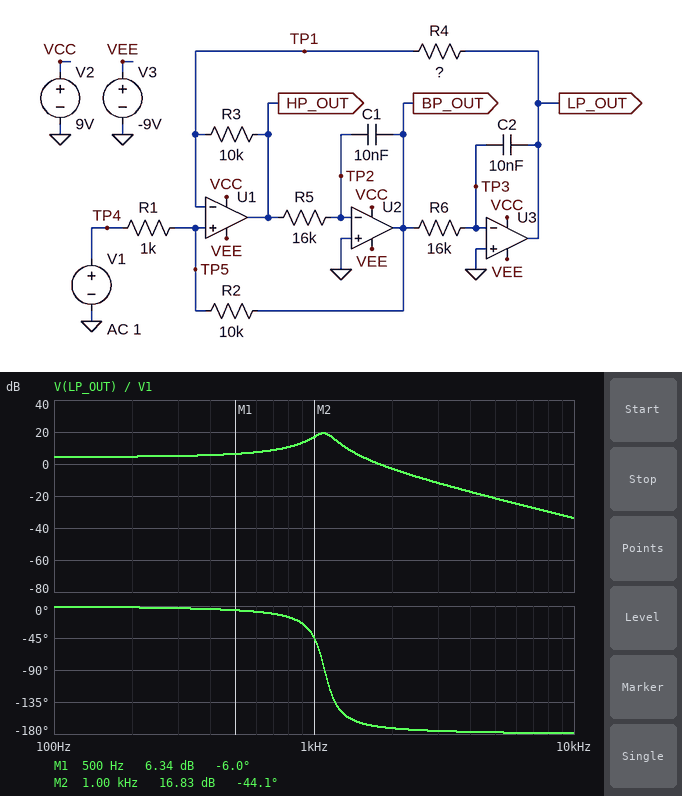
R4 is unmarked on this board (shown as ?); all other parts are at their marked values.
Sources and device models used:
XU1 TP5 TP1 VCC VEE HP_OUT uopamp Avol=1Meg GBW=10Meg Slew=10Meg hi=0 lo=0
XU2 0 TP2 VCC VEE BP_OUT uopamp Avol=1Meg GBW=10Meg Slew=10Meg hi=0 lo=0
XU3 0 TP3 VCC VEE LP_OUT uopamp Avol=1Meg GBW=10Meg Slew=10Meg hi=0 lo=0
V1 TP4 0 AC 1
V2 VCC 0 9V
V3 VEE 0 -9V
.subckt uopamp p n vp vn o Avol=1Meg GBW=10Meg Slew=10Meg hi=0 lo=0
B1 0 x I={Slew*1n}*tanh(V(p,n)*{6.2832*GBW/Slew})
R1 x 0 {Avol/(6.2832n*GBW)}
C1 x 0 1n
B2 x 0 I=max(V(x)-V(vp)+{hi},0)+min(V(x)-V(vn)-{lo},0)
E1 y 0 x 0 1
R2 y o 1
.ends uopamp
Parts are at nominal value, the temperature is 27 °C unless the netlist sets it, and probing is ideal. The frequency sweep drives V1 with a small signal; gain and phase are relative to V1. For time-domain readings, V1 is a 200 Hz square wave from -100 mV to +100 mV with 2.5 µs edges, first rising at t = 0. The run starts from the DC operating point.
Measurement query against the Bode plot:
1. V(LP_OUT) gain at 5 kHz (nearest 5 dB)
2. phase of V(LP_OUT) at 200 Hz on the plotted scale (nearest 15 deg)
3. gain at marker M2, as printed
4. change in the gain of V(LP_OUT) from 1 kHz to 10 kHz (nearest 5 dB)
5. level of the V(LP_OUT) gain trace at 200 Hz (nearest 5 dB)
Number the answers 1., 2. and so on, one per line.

1. -20 dB
2. 0 deg
3. 16.83 dB
4. -50 dB
5. 5 dB
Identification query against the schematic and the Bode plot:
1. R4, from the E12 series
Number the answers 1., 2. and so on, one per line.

1. 8.2 kΩ
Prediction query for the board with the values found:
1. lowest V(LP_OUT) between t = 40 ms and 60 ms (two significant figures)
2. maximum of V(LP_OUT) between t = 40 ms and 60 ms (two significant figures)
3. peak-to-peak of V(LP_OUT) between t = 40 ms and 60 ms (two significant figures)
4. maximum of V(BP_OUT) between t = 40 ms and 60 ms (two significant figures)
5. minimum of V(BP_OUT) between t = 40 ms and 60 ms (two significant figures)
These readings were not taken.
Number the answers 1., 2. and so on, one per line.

1. -420 mV
2. 420 mV
3. 840 mV
4. 330 mV
5. -330 mV
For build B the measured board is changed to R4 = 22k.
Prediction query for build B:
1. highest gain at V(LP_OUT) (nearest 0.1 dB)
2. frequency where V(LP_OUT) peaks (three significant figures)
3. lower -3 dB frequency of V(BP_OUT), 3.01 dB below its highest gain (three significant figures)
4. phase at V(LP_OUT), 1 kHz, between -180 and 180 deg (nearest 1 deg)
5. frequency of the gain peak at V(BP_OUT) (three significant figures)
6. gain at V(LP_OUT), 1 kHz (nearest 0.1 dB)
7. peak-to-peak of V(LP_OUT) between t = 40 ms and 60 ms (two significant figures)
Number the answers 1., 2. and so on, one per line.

1. 23.5 dB
2. 664 Hz
3. 608 Hz
4. -167 deg
5. 671 Hz
6. 7.3 dB
7. 1.6 V
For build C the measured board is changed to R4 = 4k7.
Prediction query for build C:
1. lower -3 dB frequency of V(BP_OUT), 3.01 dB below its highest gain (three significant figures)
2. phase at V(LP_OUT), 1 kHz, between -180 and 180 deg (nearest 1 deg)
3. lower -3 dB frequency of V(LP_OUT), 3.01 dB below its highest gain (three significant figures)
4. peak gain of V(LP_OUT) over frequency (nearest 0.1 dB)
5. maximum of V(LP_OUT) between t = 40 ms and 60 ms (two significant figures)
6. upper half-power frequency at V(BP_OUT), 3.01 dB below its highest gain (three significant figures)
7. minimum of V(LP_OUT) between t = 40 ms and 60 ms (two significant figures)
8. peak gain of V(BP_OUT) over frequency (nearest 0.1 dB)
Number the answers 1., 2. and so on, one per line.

1. 1.32 kHz
2. -14 deg
3. 1.29 kHz
4. 16.8 dB
5. 350 mV
6. 1.60 kHz
7. -350 mV
8. 20.0 dB
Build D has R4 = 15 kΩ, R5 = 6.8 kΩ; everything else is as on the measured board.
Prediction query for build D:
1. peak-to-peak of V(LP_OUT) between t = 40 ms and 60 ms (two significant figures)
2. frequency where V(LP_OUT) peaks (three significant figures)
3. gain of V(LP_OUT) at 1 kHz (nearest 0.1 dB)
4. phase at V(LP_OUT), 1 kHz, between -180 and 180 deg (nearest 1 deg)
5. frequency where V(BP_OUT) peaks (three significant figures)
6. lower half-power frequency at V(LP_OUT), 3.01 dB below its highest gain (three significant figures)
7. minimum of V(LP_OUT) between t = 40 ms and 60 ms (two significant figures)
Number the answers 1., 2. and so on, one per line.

1. 1.0 V
2. 1.22 kHz
3. 14.6 dB
4. -33 deg
5. 1.25 kHz
6. 1.03 kHz
7. -500 mV
